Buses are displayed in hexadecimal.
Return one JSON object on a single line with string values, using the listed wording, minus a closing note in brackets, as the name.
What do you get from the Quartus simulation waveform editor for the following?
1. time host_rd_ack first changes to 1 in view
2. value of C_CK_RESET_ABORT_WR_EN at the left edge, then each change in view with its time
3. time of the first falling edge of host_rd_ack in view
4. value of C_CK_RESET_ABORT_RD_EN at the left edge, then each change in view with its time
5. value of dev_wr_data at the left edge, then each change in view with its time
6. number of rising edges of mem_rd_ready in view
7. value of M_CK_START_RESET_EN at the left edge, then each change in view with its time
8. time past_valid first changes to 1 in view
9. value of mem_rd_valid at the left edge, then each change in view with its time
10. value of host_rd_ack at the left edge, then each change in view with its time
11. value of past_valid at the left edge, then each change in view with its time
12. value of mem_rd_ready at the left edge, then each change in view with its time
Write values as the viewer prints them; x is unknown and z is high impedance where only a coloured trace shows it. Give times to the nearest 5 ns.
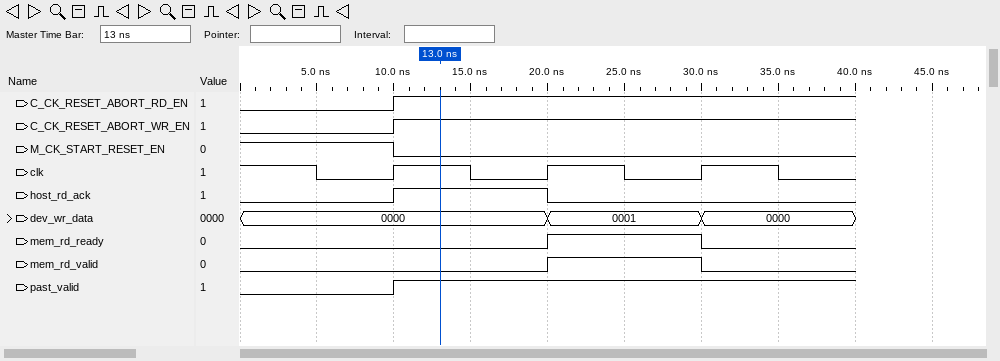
{"time host_rd_ack first changes to 1 in view": "10 ns", "value of C_CK_RESET_ABORT_WR_EN at the left edge, then each change in view with its time": "0, 1 at 10 ns", "time of the first falling edge of host_rd_ack in view": "20 ns", "value of C_CK_RESET_ABORT_RD_EN at the left edge, then each change in view with its time": "0, 1 at 10 ns", "value of dev_wr_data at the left edge, then each change in view with its time": "0000, 0001 at 20 ns, 0000 at 30 ns", "number of rising edges of mem_rd_ready in view": "1", "value of M_CK_START_RESET_EN at the left edge, then each change in view with its time": "1, 0 at 10 ns", "time past_valid first changes to 1 in view": "10 ns", "value of mem_rd_valid at the left edge, then each change in view with its time": "0, 1 at 20 ns, 0 at 30 ns", "value of host_rd_ack at the left edge, then each change in view with its time": "0, 1 at 10 ns, 0 at 20 ns", "value of past_valid at the left edge, then each change in view with its time": "0, 1 at 10 ns", "value of mem_rd_ready at the left edge, then each change in view with its time": "0, 1 at 20 ns, 0 at 30 ns"}
